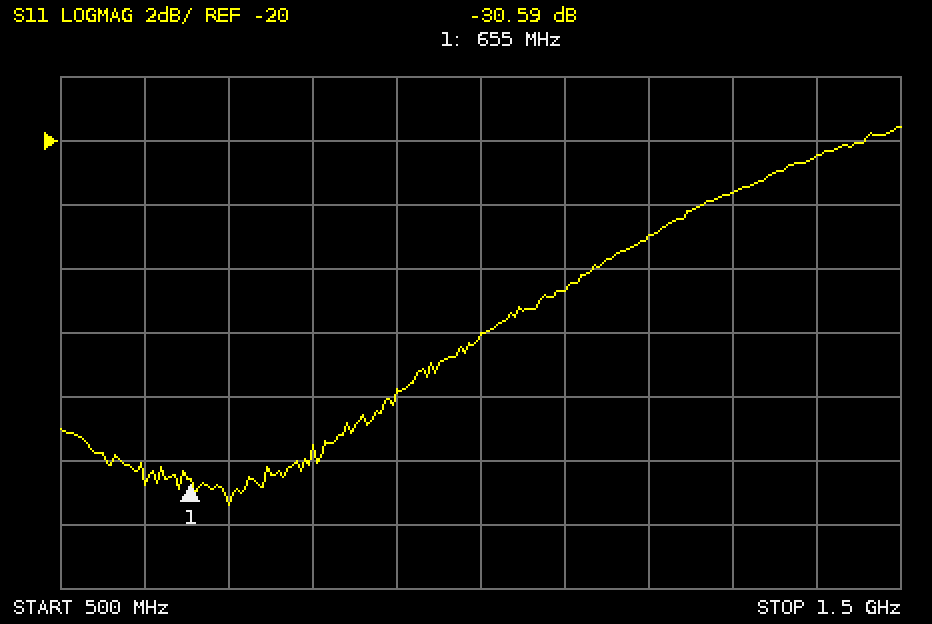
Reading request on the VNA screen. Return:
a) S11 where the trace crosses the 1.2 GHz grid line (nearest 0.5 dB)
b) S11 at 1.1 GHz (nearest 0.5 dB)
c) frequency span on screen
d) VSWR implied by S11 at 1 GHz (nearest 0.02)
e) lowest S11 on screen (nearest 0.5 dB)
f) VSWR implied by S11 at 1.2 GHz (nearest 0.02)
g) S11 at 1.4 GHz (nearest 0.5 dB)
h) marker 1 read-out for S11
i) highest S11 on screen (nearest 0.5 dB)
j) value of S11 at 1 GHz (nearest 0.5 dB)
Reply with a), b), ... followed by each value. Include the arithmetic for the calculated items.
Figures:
a) -23.0 dB
b) -24.5 dB
c) 1 GHz
d) |Γ| = 10^(-26/20) = 0.0501; VSWR = (1 + 0.0501)/(1 − 0.0501) ≈ 1.11, so 1.10 to the nearest 0.02
e) -31.5 dB
f) |Γ| = 10^(-23/20) = 0.0708; VSWR = (1 + 0.0708)/(1 − 0.0708) ≈ 1.15, so 1.16 to the nearest 0.02
g) -20.5 dB
h) -30.59 dB
i) -19.5 dB
j) -26.0 dB
